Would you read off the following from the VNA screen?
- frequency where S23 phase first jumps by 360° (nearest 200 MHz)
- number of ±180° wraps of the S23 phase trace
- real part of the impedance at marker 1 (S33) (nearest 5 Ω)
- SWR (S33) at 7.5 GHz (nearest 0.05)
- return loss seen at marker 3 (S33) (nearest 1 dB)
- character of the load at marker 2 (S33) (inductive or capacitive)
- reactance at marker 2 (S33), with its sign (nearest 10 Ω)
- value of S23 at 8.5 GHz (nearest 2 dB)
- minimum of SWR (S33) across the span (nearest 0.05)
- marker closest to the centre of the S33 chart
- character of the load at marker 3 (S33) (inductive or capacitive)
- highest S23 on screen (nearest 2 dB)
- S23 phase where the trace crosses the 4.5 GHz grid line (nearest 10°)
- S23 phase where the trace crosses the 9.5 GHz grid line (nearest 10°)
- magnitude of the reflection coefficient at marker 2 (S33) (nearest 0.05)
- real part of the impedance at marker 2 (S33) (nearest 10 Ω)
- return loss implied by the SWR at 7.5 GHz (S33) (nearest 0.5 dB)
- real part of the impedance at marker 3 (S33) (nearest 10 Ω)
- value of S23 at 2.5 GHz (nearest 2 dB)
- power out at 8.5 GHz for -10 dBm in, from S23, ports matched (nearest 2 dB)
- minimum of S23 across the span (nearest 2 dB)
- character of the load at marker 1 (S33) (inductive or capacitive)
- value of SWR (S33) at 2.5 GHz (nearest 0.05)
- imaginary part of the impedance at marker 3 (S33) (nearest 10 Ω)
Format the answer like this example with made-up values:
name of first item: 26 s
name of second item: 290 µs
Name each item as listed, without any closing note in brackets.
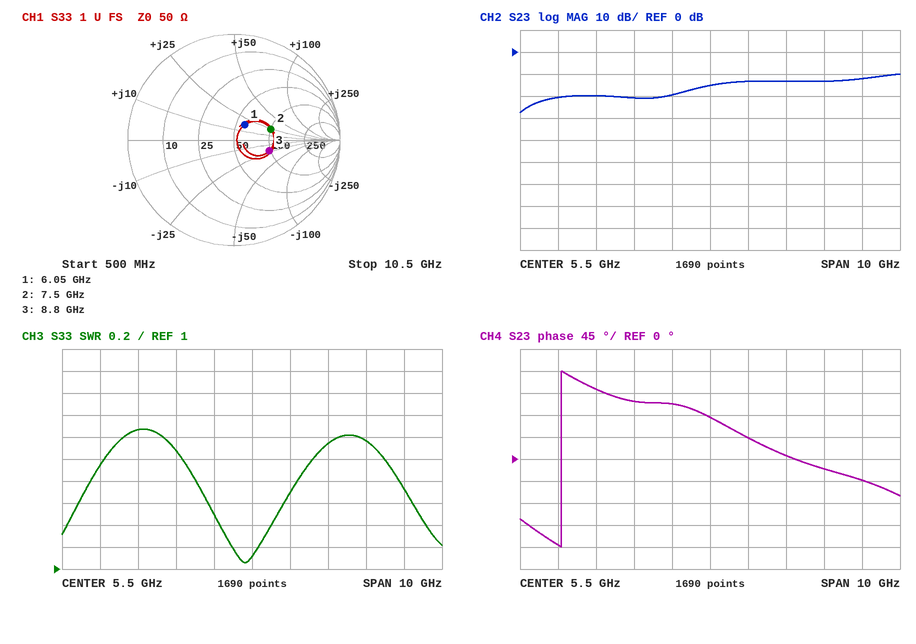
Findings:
frequency where S23 phase first jumps by 360°: 1.6 GHz
number of ±180° wraps of the S23 phase trace: 1
real part of the impedance at marker 1 (S33): 60 Ω
SWR (S33) at 7.5 GHz: 2.15
return loss seen at marker 3 (S33): 9 dB
character of the load at marker 2 (S33): inductive
reactance at marker 2 (S33), with its sign: +20 Ω
value of S23 at 8.5 GHz: -14 dB
minimum of SWR (S33) across the span: 1.05
marker closest to the centre of the S33 chart: marker 1
character of the load at marker 3 (S33): capacitive
highest S23 on screen: -10 dB
S23 phase where the trace crosses the 4.5 GHz grid line: 110°
S23 phase where the trace crosses the 9.5 GHz grid line: -40°
magnitude of the reflection coefficient at marker 2 (S33): 0.35
real part of the impedance at marker 2 (S33): 100 Ω
return loss implied by the SWR at 7.5 GHz (S33): 9.0 dB
real part of the impedance at marker 3 (S33): 100 Ω
value of S23 at 2.5 GHz: -20 dB
power out at 8.5 GHz for -10 dBm in, from S23, ports matched: -24 dBm
minimum of S23 across the span: -28 dB
character of the load at marker 1 (S33): inductive
value of SWR (S33) at 2.5 GHz: 2.25
imaginary part of the impedance at marker 3 (S33): -20 Ω
